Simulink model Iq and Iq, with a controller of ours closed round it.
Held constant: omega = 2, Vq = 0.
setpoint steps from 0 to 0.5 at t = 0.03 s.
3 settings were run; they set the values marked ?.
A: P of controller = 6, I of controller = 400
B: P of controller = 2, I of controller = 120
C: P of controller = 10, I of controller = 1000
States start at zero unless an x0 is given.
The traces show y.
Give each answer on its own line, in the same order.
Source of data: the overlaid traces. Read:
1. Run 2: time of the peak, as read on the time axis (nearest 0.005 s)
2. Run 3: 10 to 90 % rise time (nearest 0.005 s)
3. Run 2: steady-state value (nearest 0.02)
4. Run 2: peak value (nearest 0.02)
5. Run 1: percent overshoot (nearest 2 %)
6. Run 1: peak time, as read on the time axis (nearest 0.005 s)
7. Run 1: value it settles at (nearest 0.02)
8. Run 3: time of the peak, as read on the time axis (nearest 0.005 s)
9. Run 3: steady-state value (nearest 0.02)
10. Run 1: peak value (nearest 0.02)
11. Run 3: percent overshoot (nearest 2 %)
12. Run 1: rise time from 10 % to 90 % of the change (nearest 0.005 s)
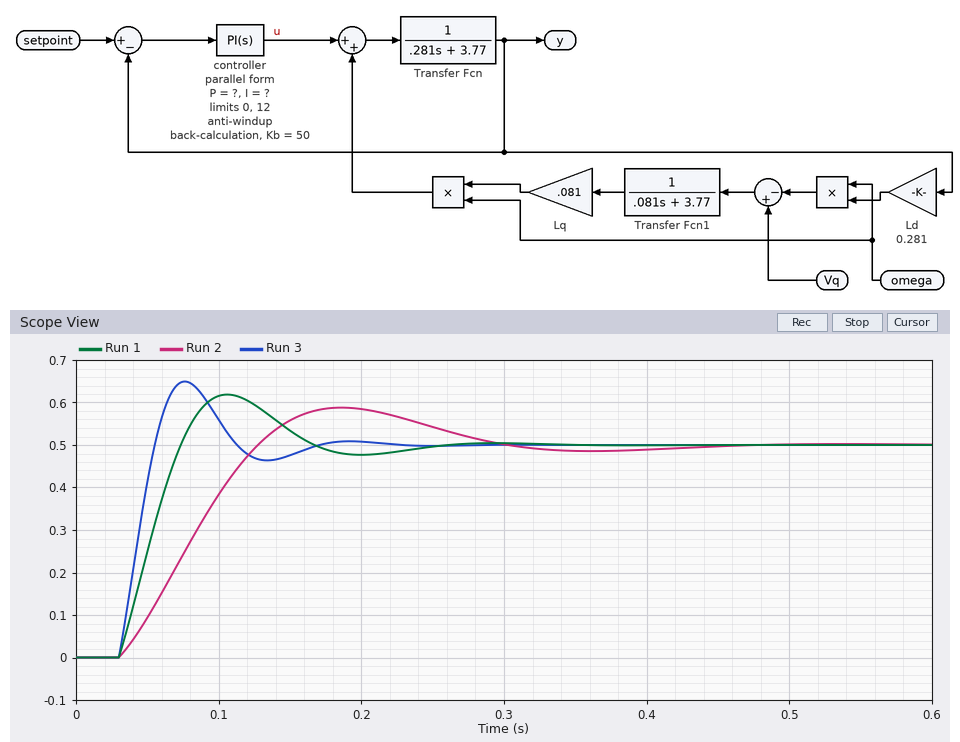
0.185 s
0.020 s
0.50
0.58
24 %
0.105 s
0.50
0.075 s
0.50
0.62
30 %
0.035 s
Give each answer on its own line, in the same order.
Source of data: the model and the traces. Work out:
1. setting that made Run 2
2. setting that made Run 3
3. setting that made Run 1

B
C
A
